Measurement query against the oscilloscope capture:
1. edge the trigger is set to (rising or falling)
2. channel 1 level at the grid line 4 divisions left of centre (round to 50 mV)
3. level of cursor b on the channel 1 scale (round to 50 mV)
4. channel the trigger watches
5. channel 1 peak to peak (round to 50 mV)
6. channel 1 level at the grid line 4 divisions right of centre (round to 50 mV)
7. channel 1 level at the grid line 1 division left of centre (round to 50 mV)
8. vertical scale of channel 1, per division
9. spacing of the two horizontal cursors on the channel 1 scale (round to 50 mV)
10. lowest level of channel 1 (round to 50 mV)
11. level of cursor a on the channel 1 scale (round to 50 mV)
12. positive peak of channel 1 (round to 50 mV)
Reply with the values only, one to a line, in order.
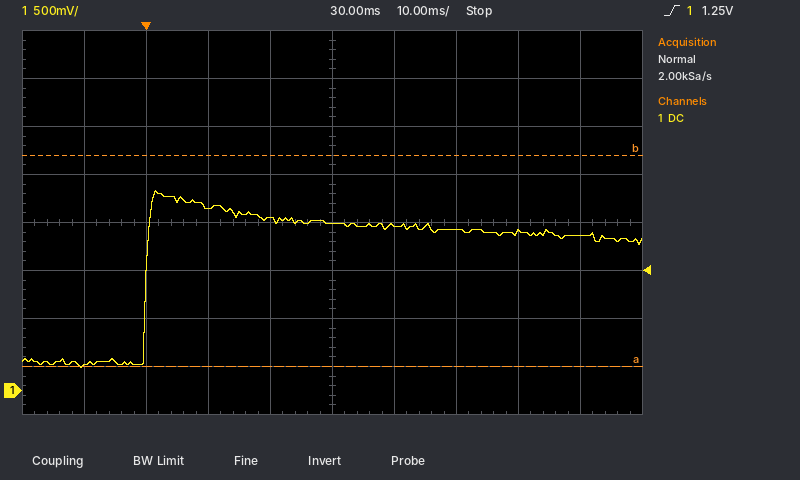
rising
250 mV
2.45 V
channel 1
1.85 V
1.60 V
1.80 V
500 mV
2.20 V
250 mV
250 mV
2.10 V
